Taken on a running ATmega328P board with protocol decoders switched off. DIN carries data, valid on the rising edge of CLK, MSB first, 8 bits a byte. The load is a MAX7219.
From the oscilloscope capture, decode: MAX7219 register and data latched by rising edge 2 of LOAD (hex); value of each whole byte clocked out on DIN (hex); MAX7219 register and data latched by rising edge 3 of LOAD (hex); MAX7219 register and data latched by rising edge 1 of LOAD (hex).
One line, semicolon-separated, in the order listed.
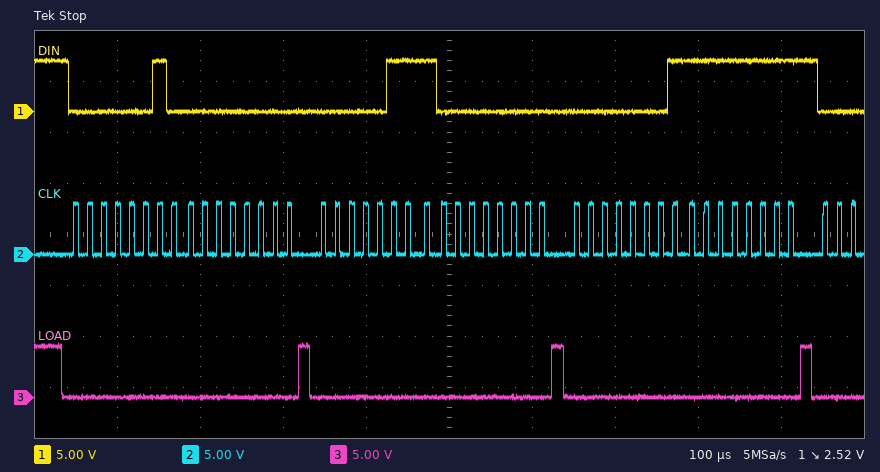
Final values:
register 0x7, data 0x00; 02 00 07 00 01 FF; register 0x1, data 0xFF; register 0x2, data 0x00
